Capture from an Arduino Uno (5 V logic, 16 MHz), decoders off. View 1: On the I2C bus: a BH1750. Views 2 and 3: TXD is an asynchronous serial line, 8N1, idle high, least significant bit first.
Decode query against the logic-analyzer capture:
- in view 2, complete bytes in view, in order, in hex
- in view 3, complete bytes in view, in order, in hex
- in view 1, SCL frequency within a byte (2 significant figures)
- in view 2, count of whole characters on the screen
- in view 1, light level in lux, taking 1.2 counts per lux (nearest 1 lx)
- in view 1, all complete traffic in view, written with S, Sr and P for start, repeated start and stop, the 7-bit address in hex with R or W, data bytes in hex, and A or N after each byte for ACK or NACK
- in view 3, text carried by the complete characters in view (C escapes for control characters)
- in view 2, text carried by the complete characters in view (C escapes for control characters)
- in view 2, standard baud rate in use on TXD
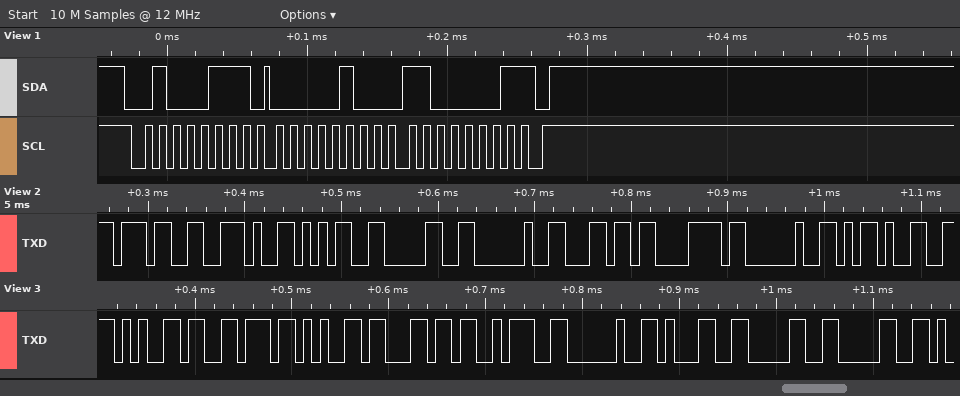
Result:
37 2E 35 30 20 6C 78 20 2D
65 76 65 6C 3A 20 31 30 30
100 kHz
9
1014 lx
S 23R A 04 A C1 N P
"evel: 100"
"7.50 lx -"
115200 baud
